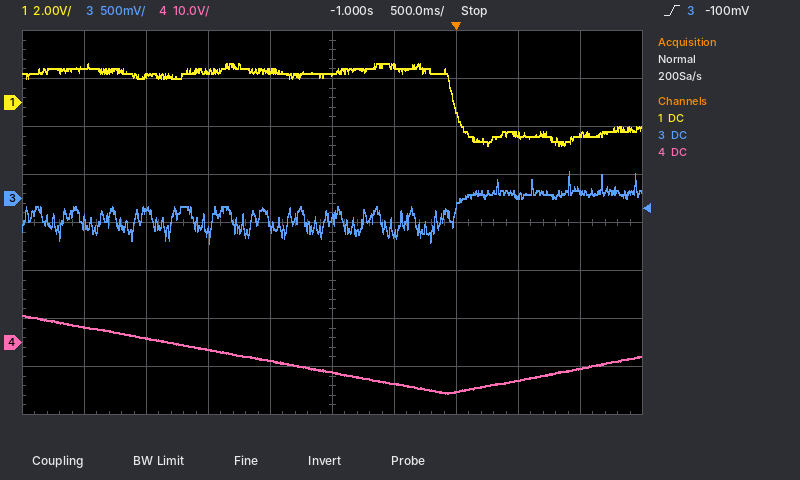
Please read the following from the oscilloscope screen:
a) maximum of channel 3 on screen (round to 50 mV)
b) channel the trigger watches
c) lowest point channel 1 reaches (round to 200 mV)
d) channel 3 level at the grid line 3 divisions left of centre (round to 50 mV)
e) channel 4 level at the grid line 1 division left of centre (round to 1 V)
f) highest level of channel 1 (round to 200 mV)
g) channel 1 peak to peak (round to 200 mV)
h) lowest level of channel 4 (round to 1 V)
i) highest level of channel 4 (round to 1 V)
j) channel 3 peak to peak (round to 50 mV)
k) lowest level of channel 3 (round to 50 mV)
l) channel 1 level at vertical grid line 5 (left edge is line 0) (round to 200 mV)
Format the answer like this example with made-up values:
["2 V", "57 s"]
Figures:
["300 mV", "channel 3", "-1.8 V", "-100 mV", "-4 V", "1.6 V", "3.4 V", "-11 V", "6 V", "750 mV", "-450 mV", "1.2 V"]
